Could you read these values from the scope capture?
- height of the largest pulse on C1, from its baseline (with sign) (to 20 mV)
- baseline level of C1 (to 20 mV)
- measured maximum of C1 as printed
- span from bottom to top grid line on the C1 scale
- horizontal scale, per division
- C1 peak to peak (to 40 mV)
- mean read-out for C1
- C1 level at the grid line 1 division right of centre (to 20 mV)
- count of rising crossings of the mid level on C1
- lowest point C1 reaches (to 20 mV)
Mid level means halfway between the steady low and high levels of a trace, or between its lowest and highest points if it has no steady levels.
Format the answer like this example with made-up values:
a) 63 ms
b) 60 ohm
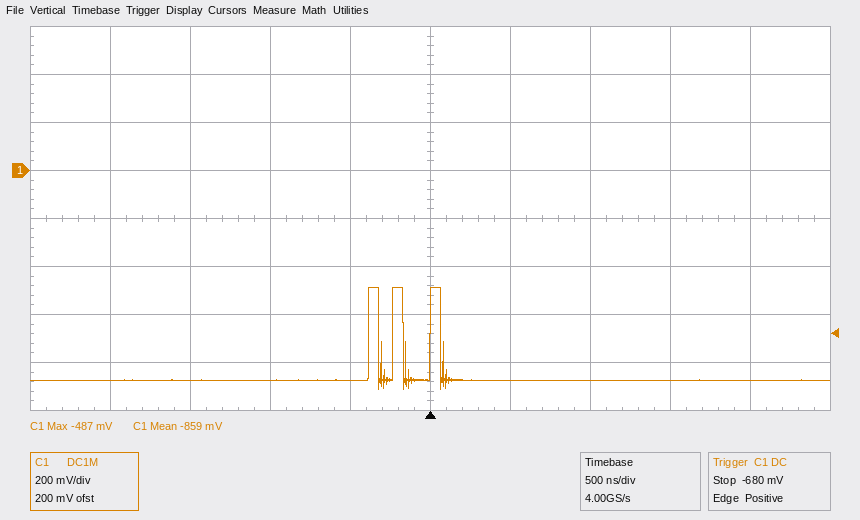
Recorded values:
a) +380 mV
b) -880 mV
c) -487 mV
d) 1.6 V
e) 500 ns
f) 440 mV
g) -859 mV
h) -880 mV
i) 3
j) -920 mV
